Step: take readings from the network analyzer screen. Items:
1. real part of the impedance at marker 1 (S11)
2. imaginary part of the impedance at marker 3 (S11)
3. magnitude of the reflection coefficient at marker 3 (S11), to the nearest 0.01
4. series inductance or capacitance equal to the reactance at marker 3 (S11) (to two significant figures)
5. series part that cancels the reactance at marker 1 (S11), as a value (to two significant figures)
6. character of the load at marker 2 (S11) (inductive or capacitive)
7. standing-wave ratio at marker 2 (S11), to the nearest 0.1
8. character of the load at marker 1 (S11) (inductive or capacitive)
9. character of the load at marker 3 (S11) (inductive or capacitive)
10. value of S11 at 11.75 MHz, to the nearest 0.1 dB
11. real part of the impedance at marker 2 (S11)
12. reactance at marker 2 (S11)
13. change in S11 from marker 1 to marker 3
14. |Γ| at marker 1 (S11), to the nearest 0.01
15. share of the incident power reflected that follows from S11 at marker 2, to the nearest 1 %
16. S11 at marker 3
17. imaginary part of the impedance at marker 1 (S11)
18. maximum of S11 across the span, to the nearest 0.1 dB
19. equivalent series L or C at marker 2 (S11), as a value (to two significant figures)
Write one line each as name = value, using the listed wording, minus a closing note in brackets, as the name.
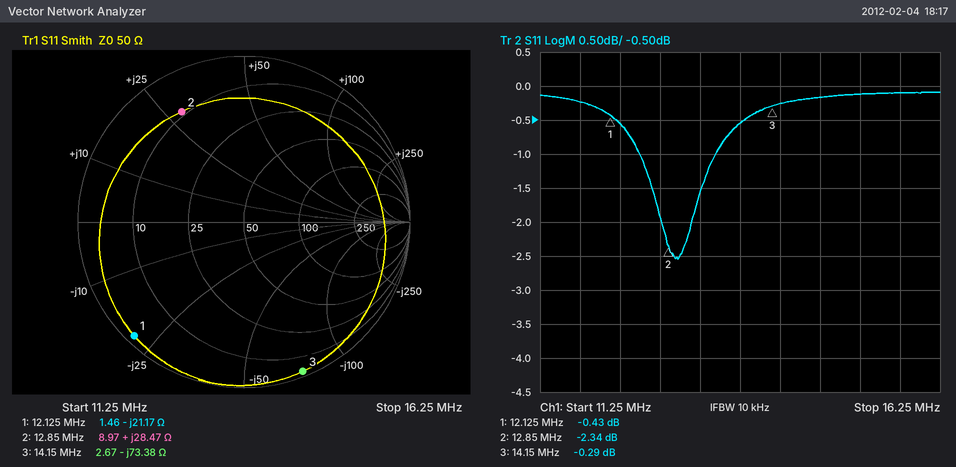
real part of the impedance at marker 1 = 1.46 Ω
imaginary part of the impedance at marker 3 = -73.38 Ω
magnitude of the reflection coefficient at marker 3 (S11), to the nearest 0.01 = 0.97
series inductance or capacitance equal to the reactance at marker 3 (S11) = 150 pF
series part that cancels the reactance at marker 1 (S11), as a value = 280 nH
character of the load at marker 2 (S11) = inductive
standing-wave ratio at marker 2 (S11), to the nearest 0.1 = 7.4
character of the load at marker 1 (S11) = capacitive
character of the load at marker 3 (S11) = capacitive
value of S11 at 11.75 MHz, to the nearest 0.1 dB = -0.2 dB
real part of the impedance at marker 2 = 8.97 Ω
reactance at marker 2 = +28.47 Ω
change in S11 from marker 1 to marker 3 = 0.14 dB
|Γ| at marker 1 (S11), to the nearest 0.01 = 0.95
share of the incident power reflected that follows from S11 at marker 2, to the nearest 1 % = 58 %
S11 at marker 3 = -0.29 dB
imaginary part of the impedance at marker 1 = -21.17 Ω
maximum of S11 across the span, to the nearest 0.1 dB = -0.1 dB
equivalent series L or C at marker 2 (S11), as a value = 350 nH
